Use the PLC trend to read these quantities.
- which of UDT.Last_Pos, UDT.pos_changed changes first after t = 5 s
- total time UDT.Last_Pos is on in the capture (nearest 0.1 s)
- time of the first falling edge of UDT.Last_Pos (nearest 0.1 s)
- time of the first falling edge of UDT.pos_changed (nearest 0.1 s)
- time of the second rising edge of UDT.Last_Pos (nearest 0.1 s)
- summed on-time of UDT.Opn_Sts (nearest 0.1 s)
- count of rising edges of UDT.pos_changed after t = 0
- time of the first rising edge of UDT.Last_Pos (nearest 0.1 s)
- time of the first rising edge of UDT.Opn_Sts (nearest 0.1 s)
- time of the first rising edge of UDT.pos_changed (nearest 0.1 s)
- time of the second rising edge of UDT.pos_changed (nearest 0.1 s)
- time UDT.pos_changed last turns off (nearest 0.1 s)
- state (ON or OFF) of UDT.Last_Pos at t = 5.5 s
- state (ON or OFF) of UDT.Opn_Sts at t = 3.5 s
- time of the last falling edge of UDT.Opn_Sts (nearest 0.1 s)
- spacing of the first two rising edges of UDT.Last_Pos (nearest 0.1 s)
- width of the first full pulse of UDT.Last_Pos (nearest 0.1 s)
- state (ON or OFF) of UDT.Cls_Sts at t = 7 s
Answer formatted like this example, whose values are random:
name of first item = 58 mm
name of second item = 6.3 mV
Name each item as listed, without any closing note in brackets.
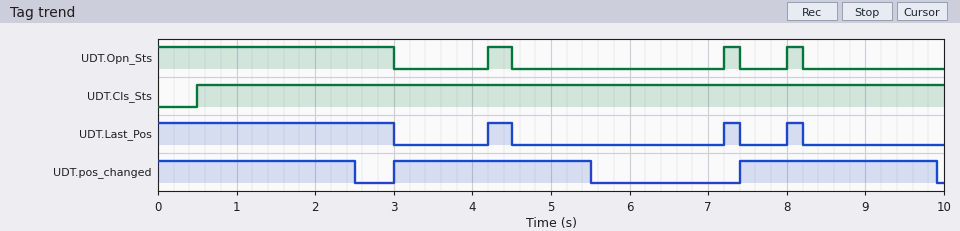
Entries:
which of UDT.Last_Pos, UDT.pos_changed changes first after t = 5 s = UDT.pos_changed
total time UDT.Last_Pos is on in the capture = 3.7 s
time of the first falling edge of UDT.Last_Pos = 3.0 s
time of the first falling edge of UDT.pos_changed = 2.5 s
time of the second rising edge of UDT.Last_Pos = 7.2 s
summed on-time of UDT.Opn_Sts = 3.7 s
count of rising edges of UDT.pos_changed after t = 0 = 2
time of the first rising edge of UDT.Last_Pos = 4.2 s
time of the first rising edge of UDT.Opn_Sts = 4.2 s
time of the first rising edge of UDT.pos_changed = 3.0 s
time of the second rising edge of UDT.pos_changed = 7.4 s
time UDT.pos_changed last turns off = 9.9 s
state (ON or OFF) of UDT.Last_Pos at t = 5.5 s = OFF
state (ON or OFF) of UDT.Opn_Sts at t = 3.5 s = OFF
time of the last falling edge of UDT.Opn_Sts = 8.2 s
spacing of the first two rising edges of UDT.Last_Pos = 3.0 s
width of the first full pulse of UDT.Last_Pos = 0.3 s
state (ON or OFF) of UDT.Cls_Sts at t = 7 s = ON
